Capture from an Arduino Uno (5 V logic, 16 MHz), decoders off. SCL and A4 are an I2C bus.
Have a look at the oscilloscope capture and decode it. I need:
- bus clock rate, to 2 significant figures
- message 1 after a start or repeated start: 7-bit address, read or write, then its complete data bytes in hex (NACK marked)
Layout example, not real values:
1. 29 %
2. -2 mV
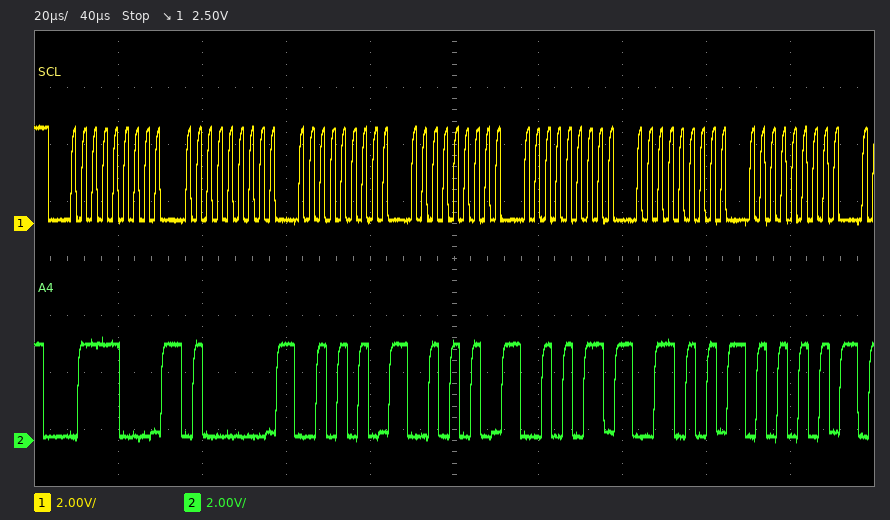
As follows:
1. 400 kHz
2. 0x3C write: 40 2A 2A 2B 35 55
